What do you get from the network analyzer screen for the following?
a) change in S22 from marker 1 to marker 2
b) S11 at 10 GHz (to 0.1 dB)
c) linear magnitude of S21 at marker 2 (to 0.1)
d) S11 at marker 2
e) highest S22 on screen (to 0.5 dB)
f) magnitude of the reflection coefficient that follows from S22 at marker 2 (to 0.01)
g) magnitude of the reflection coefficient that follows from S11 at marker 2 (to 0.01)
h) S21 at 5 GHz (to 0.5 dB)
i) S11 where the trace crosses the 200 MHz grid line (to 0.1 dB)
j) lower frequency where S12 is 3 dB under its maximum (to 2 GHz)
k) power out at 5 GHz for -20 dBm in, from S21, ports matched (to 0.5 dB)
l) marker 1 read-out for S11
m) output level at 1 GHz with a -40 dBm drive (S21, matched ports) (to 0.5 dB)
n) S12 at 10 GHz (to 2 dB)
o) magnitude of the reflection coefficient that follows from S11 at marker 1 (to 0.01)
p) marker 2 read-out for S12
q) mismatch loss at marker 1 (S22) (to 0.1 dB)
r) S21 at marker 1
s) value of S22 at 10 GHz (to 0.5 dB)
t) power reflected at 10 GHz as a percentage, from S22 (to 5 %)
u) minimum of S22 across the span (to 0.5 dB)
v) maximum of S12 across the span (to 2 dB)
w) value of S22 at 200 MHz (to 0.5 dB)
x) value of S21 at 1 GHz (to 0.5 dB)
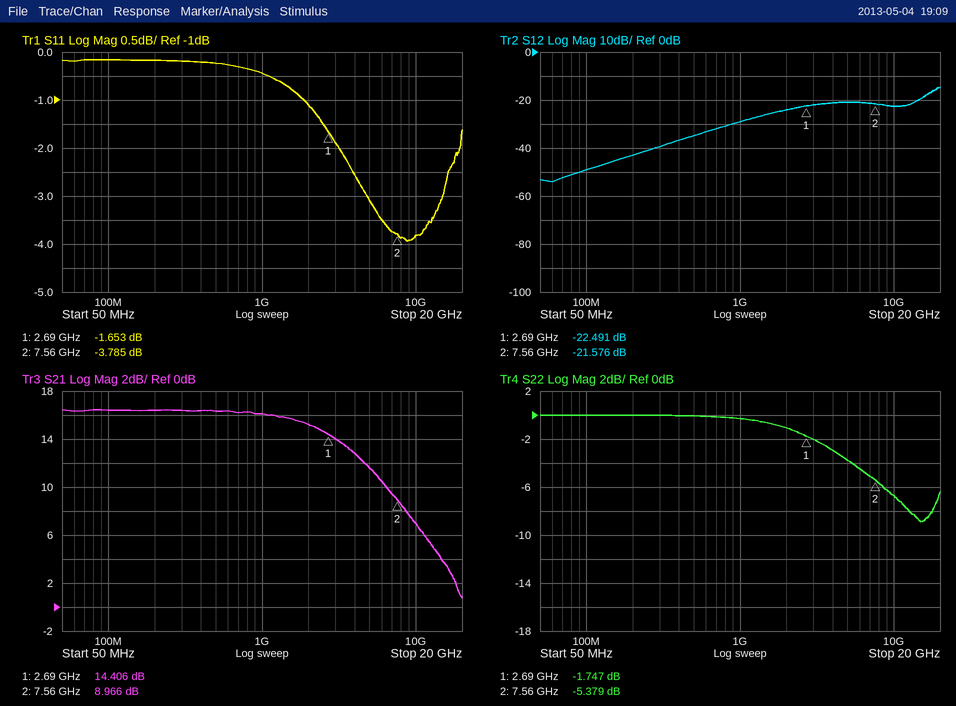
-3.632 dB
-3.8 dB
2.8
-3.785 dB
0.0 dB
0.54
0.65
11.5 dB
-0.2 dB
16 GHz
-8.5 dBm
-1.653 dB
-24.0 dBm
-22 dB
0.83
-21.576 dB
4.8 dB
14.406 dB
-6.5 dB
20 %
-9.0 dB
-14 dB
0.0 dB
16.0 dB
